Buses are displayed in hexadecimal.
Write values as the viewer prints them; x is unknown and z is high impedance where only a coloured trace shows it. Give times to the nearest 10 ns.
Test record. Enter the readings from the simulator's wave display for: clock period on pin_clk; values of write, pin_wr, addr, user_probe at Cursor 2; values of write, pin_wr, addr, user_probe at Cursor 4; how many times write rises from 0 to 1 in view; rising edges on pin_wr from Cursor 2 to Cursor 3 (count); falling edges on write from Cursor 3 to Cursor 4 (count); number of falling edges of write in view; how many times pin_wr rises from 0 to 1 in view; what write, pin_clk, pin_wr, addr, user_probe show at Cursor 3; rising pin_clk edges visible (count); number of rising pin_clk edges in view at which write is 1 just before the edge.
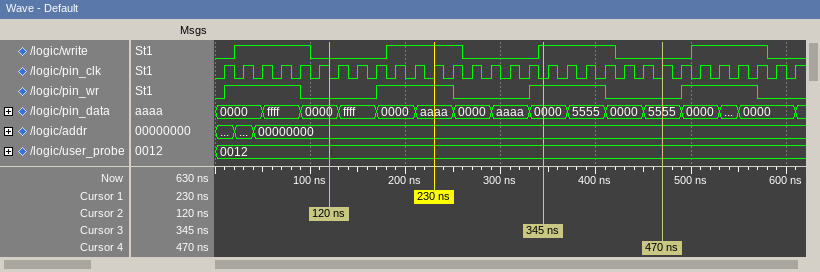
20 ns
write=0, pin_wr=0, addr=00000000, user_probe=0012
write=0, pin_wr=0, addr=00000000, user_probe=0012
4
2
1
4
4
write=1, pin_clk=0, pin_wr=1, addr=00000000, user_probe=0012
31
16
